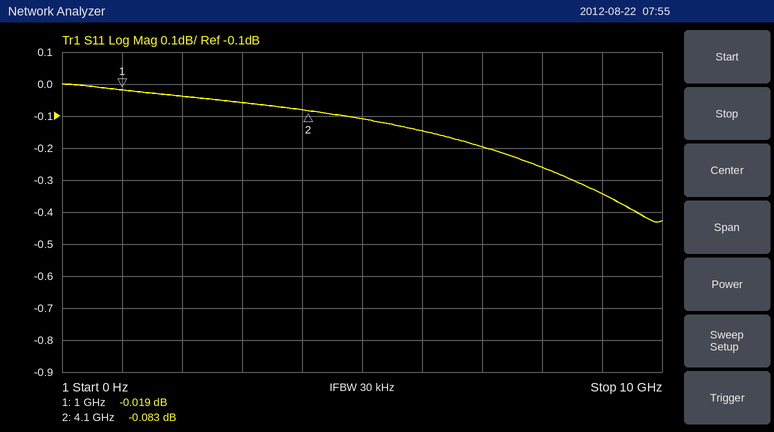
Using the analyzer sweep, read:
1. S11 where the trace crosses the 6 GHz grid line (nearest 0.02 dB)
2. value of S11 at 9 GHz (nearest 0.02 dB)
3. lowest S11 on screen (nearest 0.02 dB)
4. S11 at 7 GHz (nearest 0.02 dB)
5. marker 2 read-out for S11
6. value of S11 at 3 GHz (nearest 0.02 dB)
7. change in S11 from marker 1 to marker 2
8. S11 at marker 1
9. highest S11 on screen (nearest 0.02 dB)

-0.14 dB
-0.34 dB
-0.44 dB
-0.20 dB
-0.083 dB
-0.06 dB
-0.064 dB
-0.019 dB
0.00 dB
